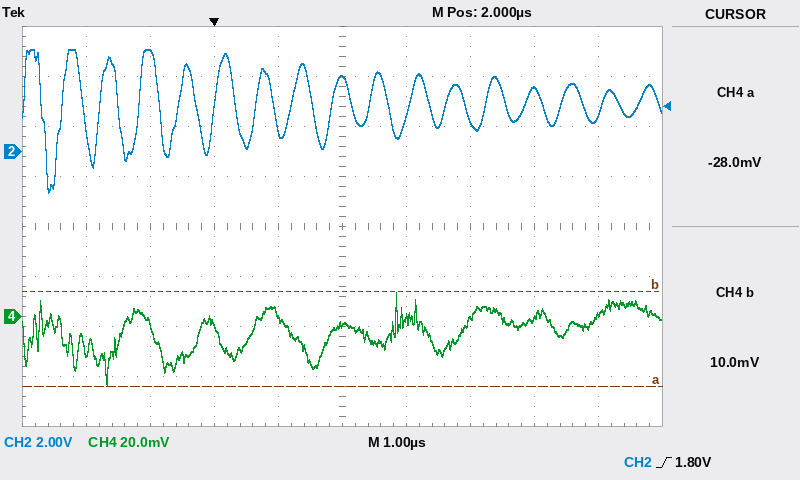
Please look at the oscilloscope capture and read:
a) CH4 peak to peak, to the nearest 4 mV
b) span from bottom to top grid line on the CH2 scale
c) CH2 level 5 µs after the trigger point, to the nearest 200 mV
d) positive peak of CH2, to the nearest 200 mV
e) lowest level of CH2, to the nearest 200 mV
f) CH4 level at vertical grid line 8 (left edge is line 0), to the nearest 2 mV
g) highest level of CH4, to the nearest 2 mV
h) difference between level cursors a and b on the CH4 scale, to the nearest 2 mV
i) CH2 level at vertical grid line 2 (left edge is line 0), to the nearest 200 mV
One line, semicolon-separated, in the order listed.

36 mV; 16 V; 2.6 V; 4.0 V; -1.6 V; 0 mV; 10 mV; 38 mV; 4.0 V
